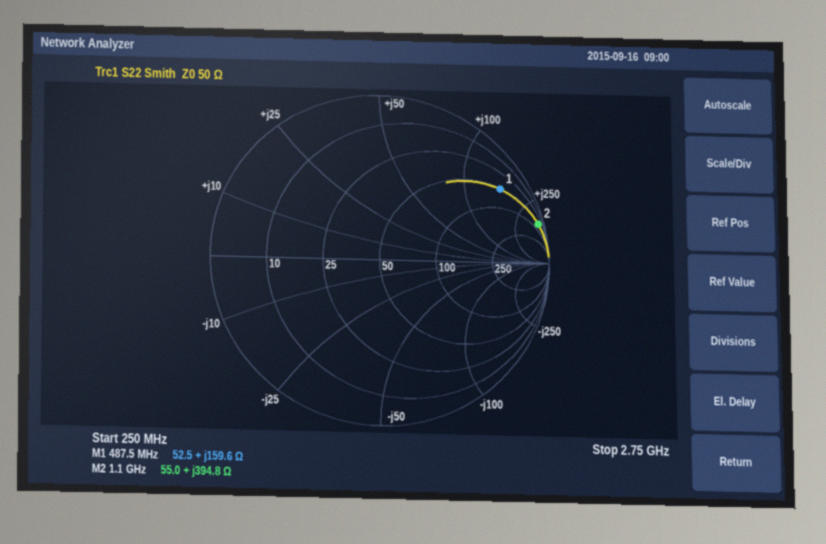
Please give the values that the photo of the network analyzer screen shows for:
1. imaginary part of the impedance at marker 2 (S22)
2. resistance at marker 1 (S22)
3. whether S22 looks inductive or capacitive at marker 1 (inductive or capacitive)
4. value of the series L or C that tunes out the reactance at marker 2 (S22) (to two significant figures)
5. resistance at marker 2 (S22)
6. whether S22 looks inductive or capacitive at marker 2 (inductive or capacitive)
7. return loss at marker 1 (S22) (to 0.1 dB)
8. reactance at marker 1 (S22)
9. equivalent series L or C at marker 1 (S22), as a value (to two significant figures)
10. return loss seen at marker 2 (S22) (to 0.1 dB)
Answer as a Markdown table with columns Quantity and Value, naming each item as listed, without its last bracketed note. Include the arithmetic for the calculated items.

| Quantity | Value |
|---|---|
| imaginary part of the impedance at marker 2 | +394.8 Ω |
| resistance at marker 1 | 52.5 Ω |
| whether S22 looks inductive or capacitive at marker 1 | inductive |
| value of the series L or C that tunes out the reactance at marker 2 (S22) | C = 1/(2π × 1.1 GHz × 394.8 Ω) ≈ 366 fF, so 370 fF to two significant figures |
| resistance at marker 2 | 55.0 Ω |
| whether S22 looks inductive or capacitive at marker 2 | inductive |
| return loss at marker 1 (S22) | 1.5 dB |
| reactance at marker 1 | +159.6 Ω |
| equivalent series L or C at marker 1 (S22), as a value | L = 159.6 Ω/(2π × 487.5 MHz) ≈ 52 nH |
| return loss seen at marker 2 (S22) | 0.3 dB |
